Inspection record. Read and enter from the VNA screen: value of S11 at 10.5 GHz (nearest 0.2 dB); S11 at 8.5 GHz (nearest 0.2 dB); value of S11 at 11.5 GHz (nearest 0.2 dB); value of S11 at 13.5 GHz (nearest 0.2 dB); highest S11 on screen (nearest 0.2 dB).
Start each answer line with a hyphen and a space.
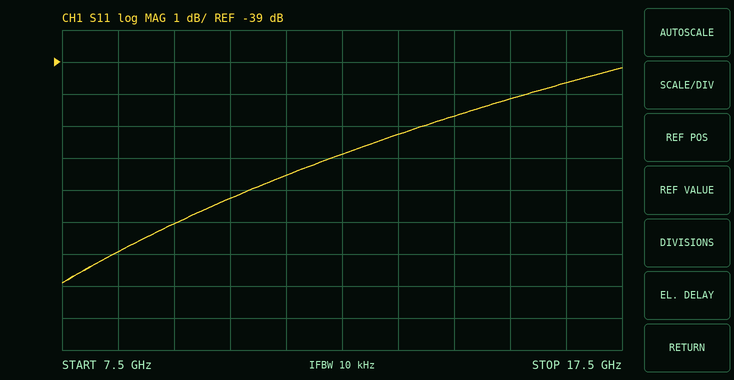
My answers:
- -43.2 dB
- -45.0 dB
- -42.6 dB
- -41.2 dB
- -39.2 dB
